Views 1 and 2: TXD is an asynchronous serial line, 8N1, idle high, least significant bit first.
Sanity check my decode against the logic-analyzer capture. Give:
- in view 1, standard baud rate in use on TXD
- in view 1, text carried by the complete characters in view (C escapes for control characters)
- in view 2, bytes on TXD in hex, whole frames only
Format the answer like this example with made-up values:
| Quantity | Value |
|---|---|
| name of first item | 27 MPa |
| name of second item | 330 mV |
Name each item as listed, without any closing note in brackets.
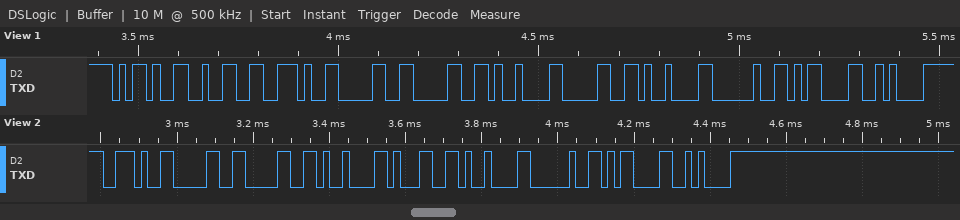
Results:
| Quantity | Value |
|---|---|
| in view 1, standard baud rate in use on TXD | 57600 baud |
| in view 1, text carried by the complete characters in view | "-2.00\t0\t \r\n" |
| in view 2, bytes on TXD in hex, whole frames only | 2E 30 30 09 31 09 20 0D 0A |
